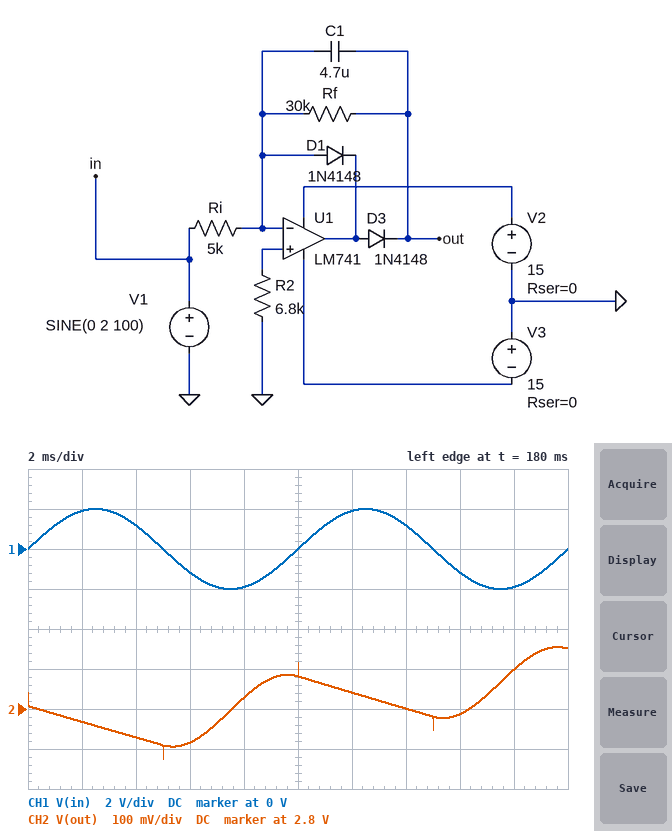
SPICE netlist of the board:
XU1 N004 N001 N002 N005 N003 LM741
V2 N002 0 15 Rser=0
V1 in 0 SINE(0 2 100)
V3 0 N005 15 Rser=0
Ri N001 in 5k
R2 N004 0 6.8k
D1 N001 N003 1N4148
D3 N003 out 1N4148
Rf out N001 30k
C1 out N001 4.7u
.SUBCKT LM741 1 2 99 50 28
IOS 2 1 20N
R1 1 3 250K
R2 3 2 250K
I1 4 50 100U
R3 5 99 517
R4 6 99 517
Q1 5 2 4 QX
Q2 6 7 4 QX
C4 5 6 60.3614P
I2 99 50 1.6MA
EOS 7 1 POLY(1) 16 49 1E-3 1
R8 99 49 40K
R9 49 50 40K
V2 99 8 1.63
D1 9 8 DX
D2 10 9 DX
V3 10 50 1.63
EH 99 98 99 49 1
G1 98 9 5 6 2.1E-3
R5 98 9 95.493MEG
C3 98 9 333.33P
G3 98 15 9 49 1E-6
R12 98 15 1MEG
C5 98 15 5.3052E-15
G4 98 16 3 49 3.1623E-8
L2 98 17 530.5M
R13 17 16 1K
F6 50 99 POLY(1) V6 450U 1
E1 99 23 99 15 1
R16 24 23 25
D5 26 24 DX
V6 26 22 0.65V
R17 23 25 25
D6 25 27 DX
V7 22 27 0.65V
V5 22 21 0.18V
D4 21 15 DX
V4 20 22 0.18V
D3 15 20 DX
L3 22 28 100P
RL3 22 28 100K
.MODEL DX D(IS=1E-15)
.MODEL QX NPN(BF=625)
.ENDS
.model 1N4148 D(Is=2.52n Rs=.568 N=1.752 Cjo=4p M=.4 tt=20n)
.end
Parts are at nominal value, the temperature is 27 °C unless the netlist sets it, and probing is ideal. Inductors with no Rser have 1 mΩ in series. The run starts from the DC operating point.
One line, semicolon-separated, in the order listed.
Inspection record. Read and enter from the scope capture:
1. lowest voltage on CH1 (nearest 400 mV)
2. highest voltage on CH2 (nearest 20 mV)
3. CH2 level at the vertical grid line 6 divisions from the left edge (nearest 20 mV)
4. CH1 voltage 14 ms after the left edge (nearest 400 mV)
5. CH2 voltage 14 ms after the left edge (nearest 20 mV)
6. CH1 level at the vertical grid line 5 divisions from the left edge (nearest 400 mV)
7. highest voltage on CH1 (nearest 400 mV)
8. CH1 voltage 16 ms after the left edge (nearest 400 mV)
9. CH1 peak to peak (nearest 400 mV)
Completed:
-2.0 V; 2.96 V; 2.84 V; 1.2 V; 2.80 V; 0 V; 2.0 V; -1.2 V; 4.0 V
